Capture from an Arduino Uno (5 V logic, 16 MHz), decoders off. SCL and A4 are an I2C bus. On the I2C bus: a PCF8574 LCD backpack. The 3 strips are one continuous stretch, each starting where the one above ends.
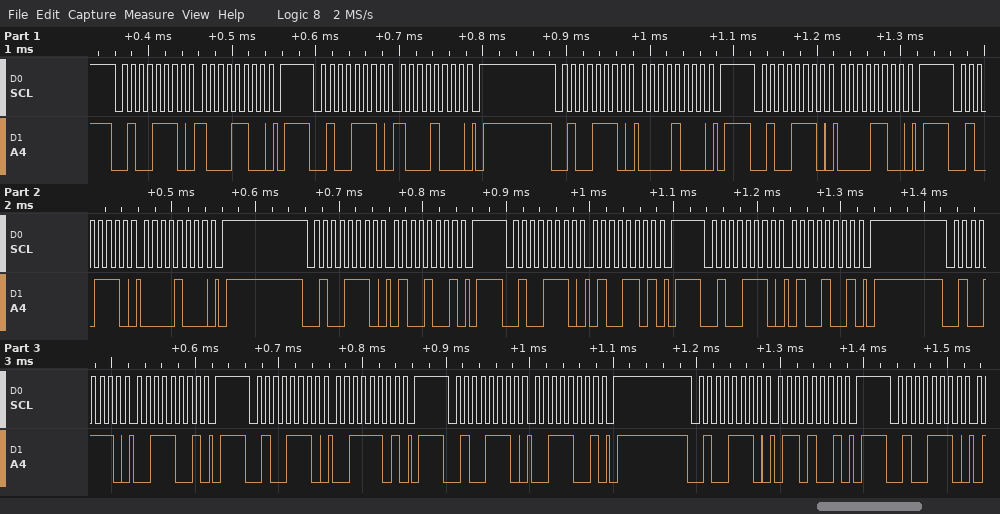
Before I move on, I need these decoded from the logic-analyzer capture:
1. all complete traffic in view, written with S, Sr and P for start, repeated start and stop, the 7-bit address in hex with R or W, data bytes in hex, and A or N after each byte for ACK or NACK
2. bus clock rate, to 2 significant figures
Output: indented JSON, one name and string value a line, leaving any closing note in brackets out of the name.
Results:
{
  "all complete traffic in view, written with S, Sr and P for start, repeated start and stop, the 7-bit address in hex with R or W, data bytes in hex, and A or N after each byte for ACK or NACK": "S 27W A 8C A P S 27W A 88 A P S 27W A 08 A P S 27W A 0C A P S 27W A 08 A P S 27W A 49 A P S 27W A 4D A P S 27W A 49 A P S 27W A 39 A P S 27W A 3D A P S 27W A 39 A P S 27W A 69 A P S 27W A",
  "bus clock rate, to 2 significant figures": "100 kHz"
}
